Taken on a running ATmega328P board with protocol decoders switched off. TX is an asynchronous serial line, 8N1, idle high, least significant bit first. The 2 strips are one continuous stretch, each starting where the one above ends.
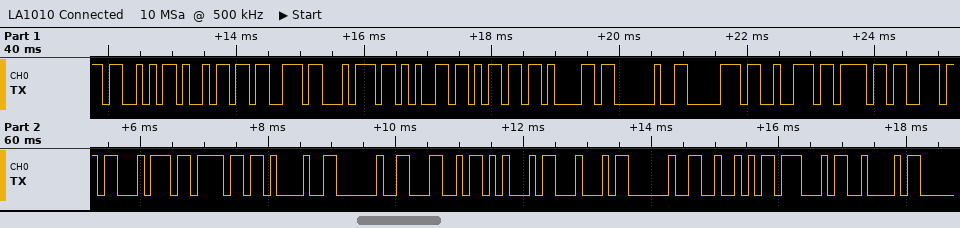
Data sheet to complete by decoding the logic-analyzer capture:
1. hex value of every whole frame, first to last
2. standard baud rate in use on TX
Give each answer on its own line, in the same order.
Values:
53 69 73 74 65 6D 61 20 70 72 6F 6E 74 6F 21 20 4C 45 44 20 52 47 42
9600 baud
